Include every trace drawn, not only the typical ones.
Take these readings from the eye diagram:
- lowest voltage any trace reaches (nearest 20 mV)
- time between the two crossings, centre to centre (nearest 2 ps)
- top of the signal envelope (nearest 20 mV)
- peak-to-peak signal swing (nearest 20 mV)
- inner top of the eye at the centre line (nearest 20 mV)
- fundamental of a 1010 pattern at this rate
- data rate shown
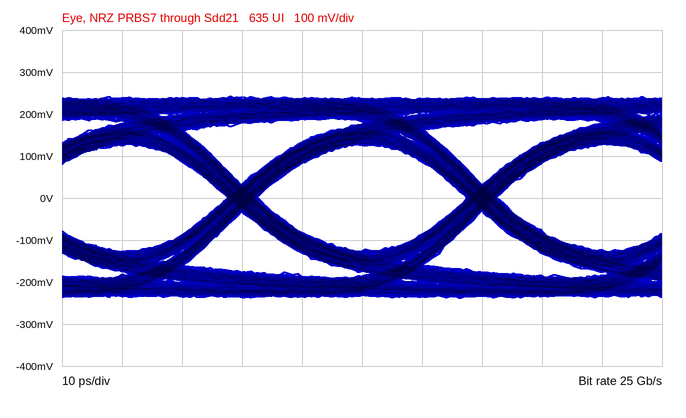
-240 mV
40 ps
240 mV
480 mV
120 mV
12.5 GHz
25 Gb/s
